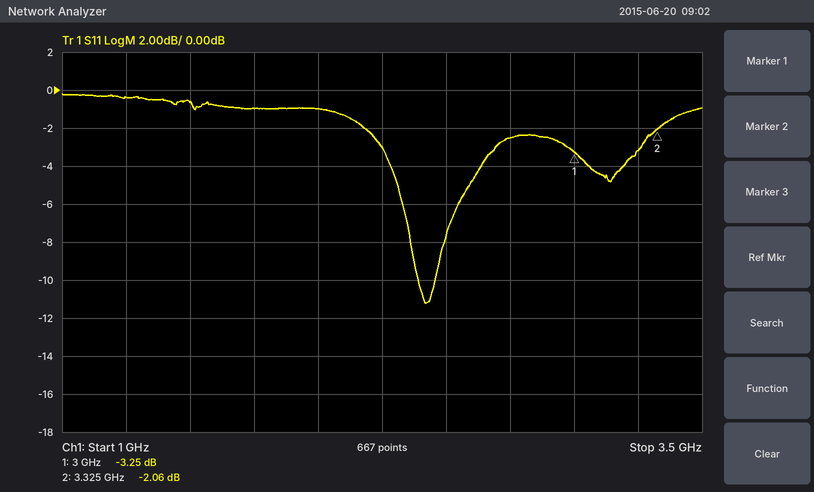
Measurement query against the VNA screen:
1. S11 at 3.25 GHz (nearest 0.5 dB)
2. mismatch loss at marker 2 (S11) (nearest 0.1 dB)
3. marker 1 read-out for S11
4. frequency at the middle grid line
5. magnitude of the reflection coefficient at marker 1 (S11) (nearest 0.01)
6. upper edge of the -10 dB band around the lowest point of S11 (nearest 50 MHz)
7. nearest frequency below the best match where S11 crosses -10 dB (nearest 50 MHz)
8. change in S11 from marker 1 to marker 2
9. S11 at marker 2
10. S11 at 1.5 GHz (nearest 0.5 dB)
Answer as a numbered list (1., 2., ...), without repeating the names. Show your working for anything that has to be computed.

1. -3.0 dB
2. −10 log10(1 − 10^(-2.06/10)) ≈ 4.2 dB
3. -3.25 dB
4. 2.25 GHz
5. 10^(-3.25/20) ≈ 0.69
6. 2.45 GHz
7. 2.40 GHz
8. -2.06 − (-3.25) = 1.19 dB
9. -2.06 dB
10. -0.5 dB
